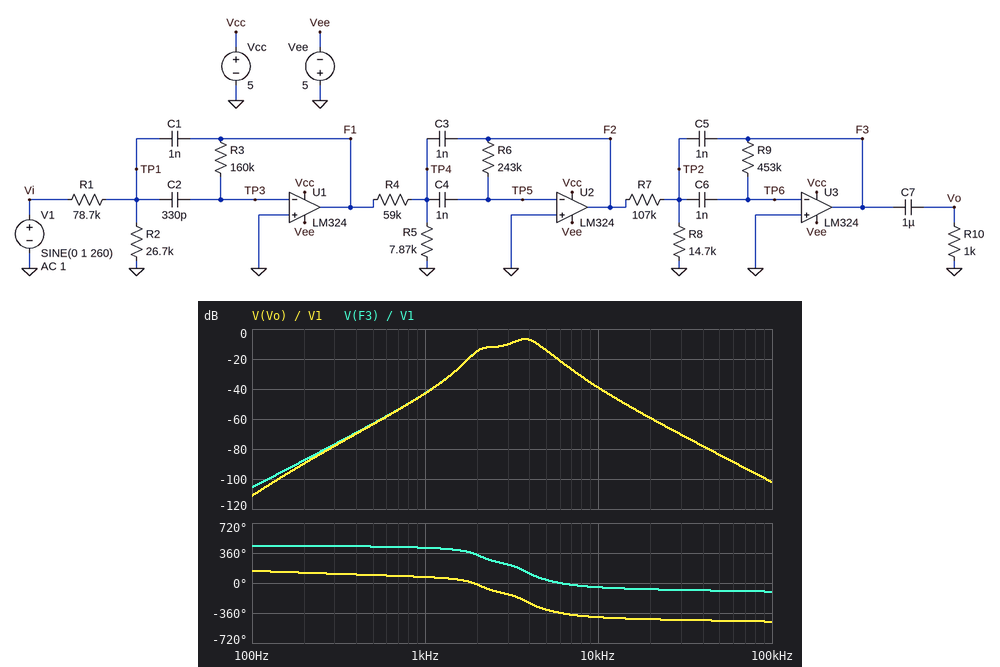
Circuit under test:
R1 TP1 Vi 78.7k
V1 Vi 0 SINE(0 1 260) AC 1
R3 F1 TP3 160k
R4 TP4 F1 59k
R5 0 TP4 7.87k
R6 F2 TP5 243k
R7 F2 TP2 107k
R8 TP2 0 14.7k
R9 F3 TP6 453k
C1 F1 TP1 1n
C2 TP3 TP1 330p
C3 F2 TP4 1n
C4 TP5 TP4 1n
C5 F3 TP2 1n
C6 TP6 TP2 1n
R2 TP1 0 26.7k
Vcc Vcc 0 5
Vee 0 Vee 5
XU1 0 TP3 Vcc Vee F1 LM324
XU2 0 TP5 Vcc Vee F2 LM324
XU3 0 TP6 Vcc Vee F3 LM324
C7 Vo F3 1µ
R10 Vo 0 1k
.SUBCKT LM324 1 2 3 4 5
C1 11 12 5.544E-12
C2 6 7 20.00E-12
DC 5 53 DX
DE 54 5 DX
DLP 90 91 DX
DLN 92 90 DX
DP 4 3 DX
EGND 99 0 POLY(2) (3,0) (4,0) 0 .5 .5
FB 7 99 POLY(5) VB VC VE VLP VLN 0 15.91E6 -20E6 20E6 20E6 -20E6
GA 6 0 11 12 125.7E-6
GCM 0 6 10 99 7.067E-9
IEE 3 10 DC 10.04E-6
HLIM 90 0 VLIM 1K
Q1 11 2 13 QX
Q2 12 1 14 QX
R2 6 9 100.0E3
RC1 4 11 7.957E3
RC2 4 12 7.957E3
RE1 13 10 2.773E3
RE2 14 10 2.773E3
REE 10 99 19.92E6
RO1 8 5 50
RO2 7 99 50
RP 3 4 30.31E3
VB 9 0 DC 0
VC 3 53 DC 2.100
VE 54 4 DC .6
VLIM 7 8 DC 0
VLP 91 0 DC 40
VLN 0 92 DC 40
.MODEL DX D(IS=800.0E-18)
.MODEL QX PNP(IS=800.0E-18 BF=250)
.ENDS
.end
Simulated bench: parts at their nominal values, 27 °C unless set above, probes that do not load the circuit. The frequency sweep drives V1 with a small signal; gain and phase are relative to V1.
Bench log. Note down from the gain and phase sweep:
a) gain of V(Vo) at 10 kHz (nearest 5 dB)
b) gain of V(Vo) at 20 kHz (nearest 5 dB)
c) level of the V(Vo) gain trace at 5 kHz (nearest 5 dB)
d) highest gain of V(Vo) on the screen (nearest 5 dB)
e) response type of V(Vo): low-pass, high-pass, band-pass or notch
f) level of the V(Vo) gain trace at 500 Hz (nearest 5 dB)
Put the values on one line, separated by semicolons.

-40 dB; -60 dB; -15 dB; -5 dB; band-pass; -65 dB
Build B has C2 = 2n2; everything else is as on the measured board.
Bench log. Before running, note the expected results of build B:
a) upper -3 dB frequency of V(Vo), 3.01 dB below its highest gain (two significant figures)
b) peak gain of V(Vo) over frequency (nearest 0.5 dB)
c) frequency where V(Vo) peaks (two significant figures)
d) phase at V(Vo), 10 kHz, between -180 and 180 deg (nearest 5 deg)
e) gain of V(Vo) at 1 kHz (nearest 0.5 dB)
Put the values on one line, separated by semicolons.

2.6 kHz; 3.5 dB; 2.1 kHz; -70 deg; -25.0 dB
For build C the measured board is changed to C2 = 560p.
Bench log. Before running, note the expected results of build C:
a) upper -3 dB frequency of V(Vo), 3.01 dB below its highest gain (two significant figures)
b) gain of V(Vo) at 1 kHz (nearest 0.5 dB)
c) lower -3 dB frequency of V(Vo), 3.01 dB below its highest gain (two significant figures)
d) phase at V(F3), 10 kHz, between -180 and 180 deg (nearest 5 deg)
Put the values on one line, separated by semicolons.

4.2 kHz; -38.0 dB; 2.9 kHz; -60 deg
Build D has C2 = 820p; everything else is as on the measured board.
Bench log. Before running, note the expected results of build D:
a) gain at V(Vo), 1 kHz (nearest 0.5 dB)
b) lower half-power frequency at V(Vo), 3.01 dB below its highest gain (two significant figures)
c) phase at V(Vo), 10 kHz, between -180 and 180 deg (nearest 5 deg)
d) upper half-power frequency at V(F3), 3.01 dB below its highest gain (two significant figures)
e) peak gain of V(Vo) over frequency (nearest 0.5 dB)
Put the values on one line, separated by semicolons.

-34.5 dB; 2.1 kHz; -65 deg; 4.0 kHz; -0.5 dB
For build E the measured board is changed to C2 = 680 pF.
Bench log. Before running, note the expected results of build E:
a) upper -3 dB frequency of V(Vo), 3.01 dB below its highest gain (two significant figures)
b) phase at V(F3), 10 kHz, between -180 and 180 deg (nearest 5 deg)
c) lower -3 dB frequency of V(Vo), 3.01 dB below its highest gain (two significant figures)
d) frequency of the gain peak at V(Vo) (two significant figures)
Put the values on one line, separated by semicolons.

4.1 kHz; -65 deg; 2.6 kHz; 3.6 kHz
